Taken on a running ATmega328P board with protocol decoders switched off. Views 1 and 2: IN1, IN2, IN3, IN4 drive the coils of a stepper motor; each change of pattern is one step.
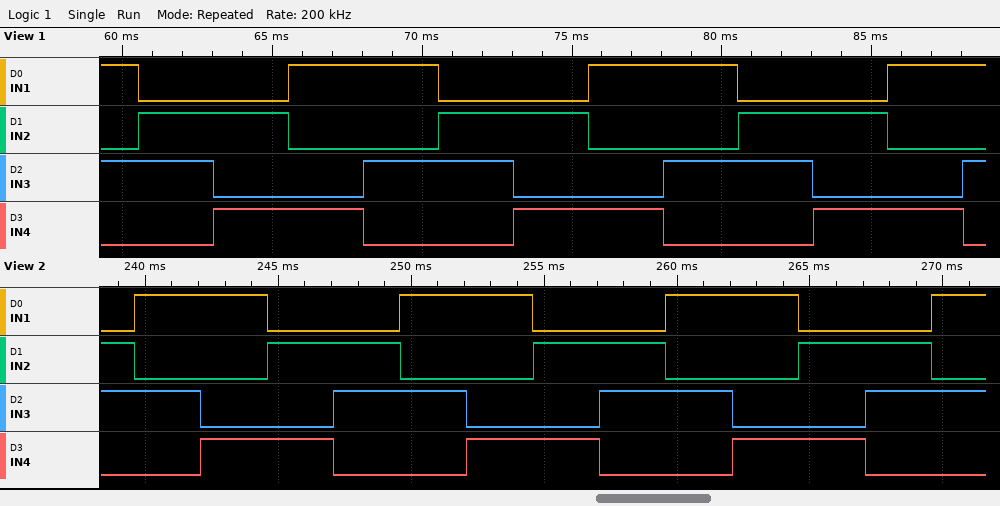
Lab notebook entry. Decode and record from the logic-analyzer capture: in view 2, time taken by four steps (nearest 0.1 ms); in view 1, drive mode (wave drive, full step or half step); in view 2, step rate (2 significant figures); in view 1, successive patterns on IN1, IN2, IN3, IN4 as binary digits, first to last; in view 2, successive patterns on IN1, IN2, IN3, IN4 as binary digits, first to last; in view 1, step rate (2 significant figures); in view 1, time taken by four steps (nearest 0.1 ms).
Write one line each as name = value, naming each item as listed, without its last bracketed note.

in view 2, time taken by four steps = 10.0 ms
in view 1, drive mode = full step
in view 2, step rate = 400 steps/s
in view 1, successive patterns on IN1, IN2, IN3, IN4 as binary digits, first to last = 1010 0110 0101 1001 1010 0110 0101 1001 1010 0110 0101 1001 1010
in view 2, successive patterns on IN1, IN2, IN3, IN4 as binary digits, first to last = 0110 1010 1001 0101 0110 1010 1001 0101 0110 1010 1001 0101 0110 1010
in view 1, step rate = 400 steps/s
in view 1, time taken by four steps = 10.0 ms
